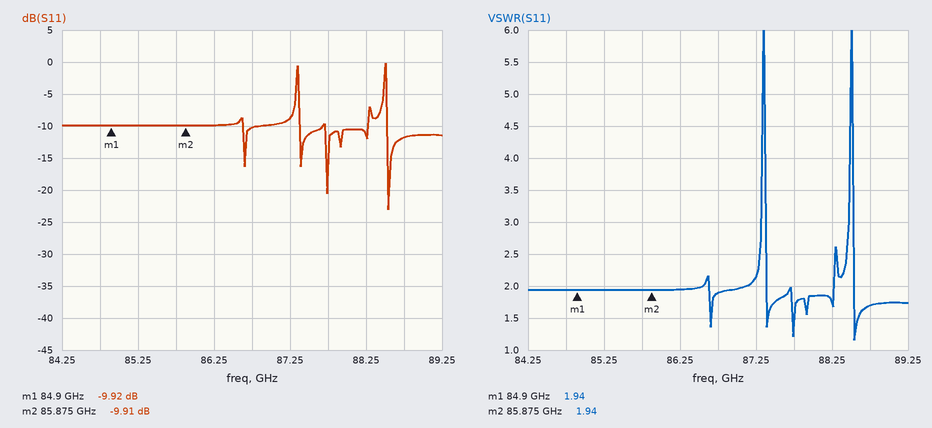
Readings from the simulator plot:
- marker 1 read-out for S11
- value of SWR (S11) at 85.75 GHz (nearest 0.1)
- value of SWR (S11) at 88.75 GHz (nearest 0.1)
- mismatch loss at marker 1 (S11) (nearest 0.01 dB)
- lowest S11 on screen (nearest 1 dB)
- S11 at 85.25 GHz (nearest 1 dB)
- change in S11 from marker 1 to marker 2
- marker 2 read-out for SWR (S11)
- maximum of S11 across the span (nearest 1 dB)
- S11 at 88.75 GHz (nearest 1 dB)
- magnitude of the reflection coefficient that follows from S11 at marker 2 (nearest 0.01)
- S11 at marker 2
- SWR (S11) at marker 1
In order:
-9.92 dB
1.9
1.7
0.47 dB
-23 dB
-10 dB
0.01 dB
1.94
0 dB
-12 dB
0.32
-9.91 dB
1.94
